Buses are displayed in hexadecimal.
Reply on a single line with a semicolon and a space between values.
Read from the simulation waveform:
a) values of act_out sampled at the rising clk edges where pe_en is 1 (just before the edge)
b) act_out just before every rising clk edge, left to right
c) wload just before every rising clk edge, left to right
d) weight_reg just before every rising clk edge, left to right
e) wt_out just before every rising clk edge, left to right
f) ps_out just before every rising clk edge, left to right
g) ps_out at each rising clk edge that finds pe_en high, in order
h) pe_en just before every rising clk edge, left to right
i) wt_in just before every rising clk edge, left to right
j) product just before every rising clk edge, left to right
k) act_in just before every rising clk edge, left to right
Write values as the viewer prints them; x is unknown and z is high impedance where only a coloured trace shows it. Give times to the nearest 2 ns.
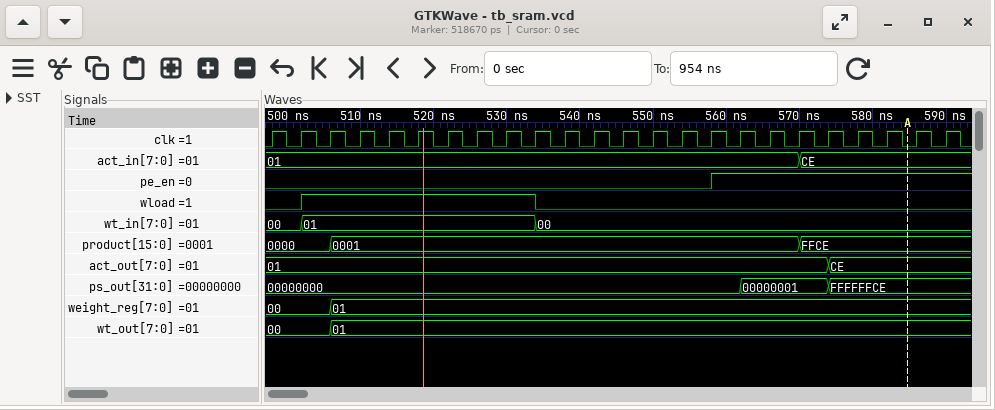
01, 01, 01, 01, CE, CE, CE, CE; 01, 01, 01, 01, 01, 01, 01, 01, 01, 01, 01, 01, 01, 01, 01, 01, 01, 01, 01, 01, CE, CE, CE, CE; 0 0 1 1 1 1 1 1 1 1 0 0 0 0 0 0 0 0 0 0 0 0 0 0; 00, 00, 00, 01, 01, 01, 01, 01, 01, 01, 01, 01, 01, 01, 01, 01, 01, 01, 01, 01, 01, 01, 01, 01; 00, 00, 00, 01, 01, 01, 01, 01, 01, 01, 01, 01, 01, 01, 01, 01, 01, 01, 01, 01, 01, 01, 01, 01; 00000000, 00000000, 00000000, 00000000, 00000000, 00000000, 00000000, 00000000, 00000000, 00000000, 00000000, 00000000, 00000000, 00000000, 00000000, 00000000, 00000000, 00000001, 00000001, 00000001, FFFFFFCE, FFFFFFCE, FFFFFFCE, FFFFFFCE; 00000000, 00000001, 00000001, 00000001, FFFFFFCE, FFFFFFCE, FFFFFFCE, FFFFFFCE; 0 0 0 0 0 0 0 0 0 0 0 0 0 0 0 0 1 1 1 1 1 1 1 1; 00, 00, 01, 01, 01, 01, 01, 01, 01, 01, 00, 00, 00, 00, 00, 00, 00, 00, 00, 00, 00, 00, 00, 00; 0000, 0000, 0000, 0001, 0001, 0001, 0001, 0001, 0001, 0001, 0001, 0001, 0001, 0001, 0001, 0001, 0001, 0001, 0001, FFCE, FFCE, FFCE, FFCE, FFCE; 01, 01, 01, 01, 01, 01, 01, 01, 01, 01, 01, 01, 01, 01, 01, 01, 01, 01, 01, CE, CE, CE, CE, CE
